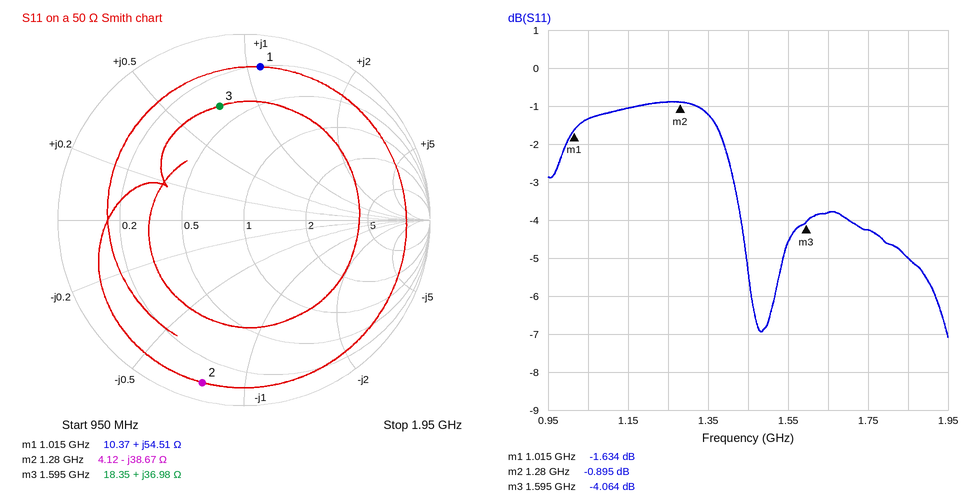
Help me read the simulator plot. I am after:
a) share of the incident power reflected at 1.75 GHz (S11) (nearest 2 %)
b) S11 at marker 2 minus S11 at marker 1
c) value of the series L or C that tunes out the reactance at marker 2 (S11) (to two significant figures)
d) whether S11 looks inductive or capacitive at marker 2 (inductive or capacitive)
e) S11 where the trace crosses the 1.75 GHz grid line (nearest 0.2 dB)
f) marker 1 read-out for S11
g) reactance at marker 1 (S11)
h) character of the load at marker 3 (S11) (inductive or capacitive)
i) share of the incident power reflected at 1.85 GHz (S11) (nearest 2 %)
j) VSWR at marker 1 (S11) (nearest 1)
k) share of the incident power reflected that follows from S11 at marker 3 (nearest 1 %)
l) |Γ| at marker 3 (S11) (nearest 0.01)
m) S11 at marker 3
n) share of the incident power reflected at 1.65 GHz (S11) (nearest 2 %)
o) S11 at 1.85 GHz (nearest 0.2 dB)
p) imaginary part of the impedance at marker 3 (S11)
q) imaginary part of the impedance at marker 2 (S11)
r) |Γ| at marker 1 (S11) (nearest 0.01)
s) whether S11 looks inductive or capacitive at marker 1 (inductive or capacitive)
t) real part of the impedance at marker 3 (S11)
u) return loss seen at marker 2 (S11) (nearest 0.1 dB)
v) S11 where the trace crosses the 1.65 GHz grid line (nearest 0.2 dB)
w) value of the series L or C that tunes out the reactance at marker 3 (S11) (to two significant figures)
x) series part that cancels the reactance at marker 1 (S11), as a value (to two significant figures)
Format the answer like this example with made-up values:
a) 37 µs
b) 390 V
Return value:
a) 38 %
b) 0.739 dB
c) 4.8 nH
d) capacitive
e) -4.2 dB
f) -1.634 dB
g) +54.51 Ω
h) inductive
i) 32 %
j) 11
k) 39 %
l) 0.63
m) -4.064 dB
n) 42 %
o) -5.0 dB
p) +36.98 Ω
q) -38.67 Ω
r) 0.83
s) inductive
t) 18.35 Ω
u) 0.9 dB
v) -3.8 dB
w) 2.7 pF
x) 2.9 pF
